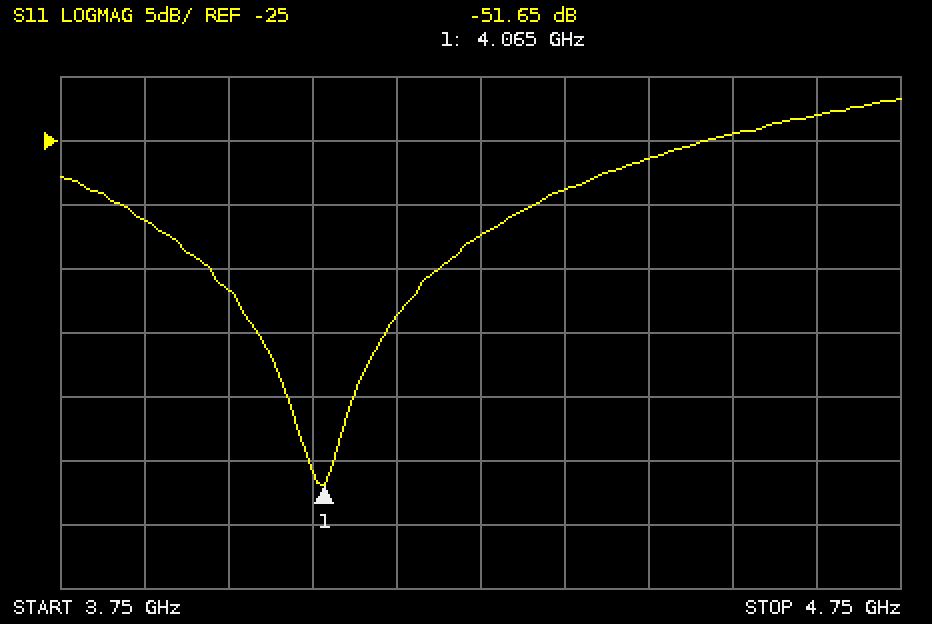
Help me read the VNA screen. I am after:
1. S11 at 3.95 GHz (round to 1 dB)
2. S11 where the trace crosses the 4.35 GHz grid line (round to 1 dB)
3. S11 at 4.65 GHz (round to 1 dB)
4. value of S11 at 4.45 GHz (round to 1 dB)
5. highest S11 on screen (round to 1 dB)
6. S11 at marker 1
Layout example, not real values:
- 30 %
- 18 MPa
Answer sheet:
- -37 dB
- -29 dB
- -23 dB
- -26 dB
- -22 dB
- -51.65 dB
